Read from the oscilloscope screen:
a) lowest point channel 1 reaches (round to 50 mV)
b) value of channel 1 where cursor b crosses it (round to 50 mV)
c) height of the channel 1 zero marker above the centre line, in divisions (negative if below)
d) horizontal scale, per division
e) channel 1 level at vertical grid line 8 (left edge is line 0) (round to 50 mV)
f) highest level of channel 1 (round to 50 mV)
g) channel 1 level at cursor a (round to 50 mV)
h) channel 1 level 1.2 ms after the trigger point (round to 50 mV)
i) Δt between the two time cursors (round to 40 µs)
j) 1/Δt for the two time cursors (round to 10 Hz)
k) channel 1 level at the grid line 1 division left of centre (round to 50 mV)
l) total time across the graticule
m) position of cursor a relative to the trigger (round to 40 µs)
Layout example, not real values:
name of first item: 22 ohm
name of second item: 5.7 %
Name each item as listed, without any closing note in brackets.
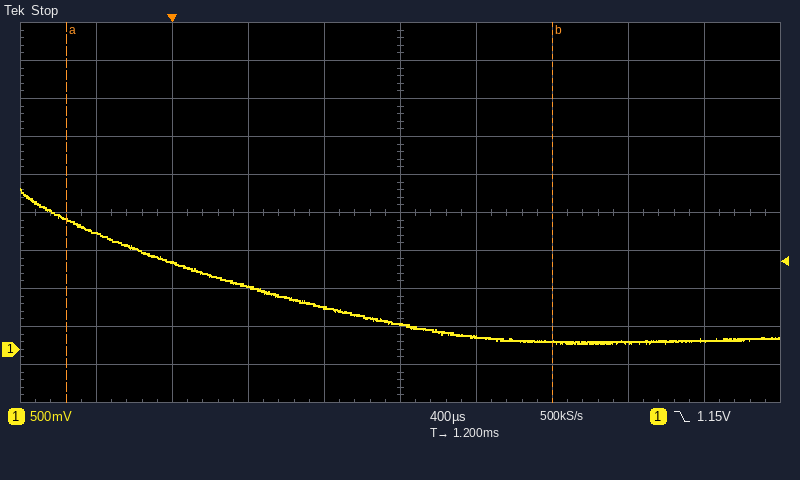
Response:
lowest point channel 1 reaches: 100 mV
value of channel 1 where cursor b crosses it: 100 mV
height of the channel 1 zero marker above the centre line, in divisions: -3.6 div
horizontal scale, per division: 400 µs
channel 1 level at vertical grid line 8 (left edge is line 0): 100 mV
highest level of channel 1: 2.10 V
channel 1 level at cursor a: 1.70 V
channel 1 level 1.2 ms after the trigger point: 350 mV
Δt between the two time cursors: 2.56 ms
1/Δt for the two time cursors: 390 Hz
channel 1 level at the grid line 1 division left of centre: 550 mV
total time across the graticule: 4 ms
position of cursor a relative to the trigger: -560 µs
